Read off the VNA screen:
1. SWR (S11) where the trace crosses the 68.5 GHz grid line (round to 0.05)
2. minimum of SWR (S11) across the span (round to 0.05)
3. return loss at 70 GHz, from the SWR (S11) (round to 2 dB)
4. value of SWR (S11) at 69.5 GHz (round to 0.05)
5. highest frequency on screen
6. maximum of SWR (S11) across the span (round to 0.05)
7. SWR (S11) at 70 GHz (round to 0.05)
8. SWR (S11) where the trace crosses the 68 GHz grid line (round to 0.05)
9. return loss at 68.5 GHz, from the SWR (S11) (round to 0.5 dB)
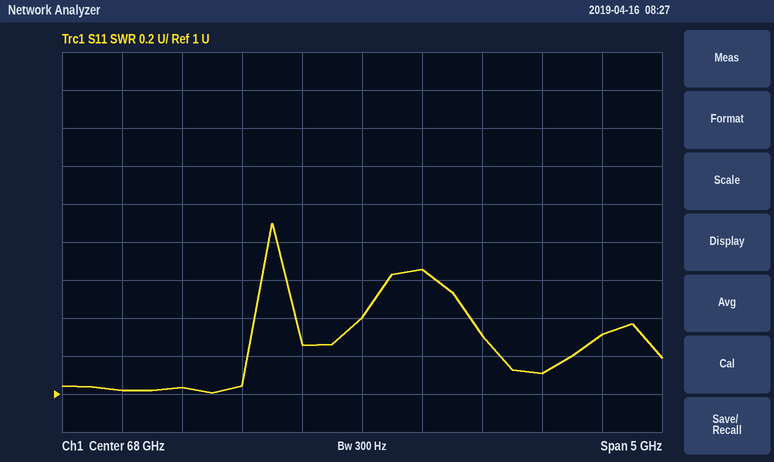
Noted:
1.65
1.00
18 dB
1.10
70.5 GHz
1.90
1.30
1.40
12.0 dB
